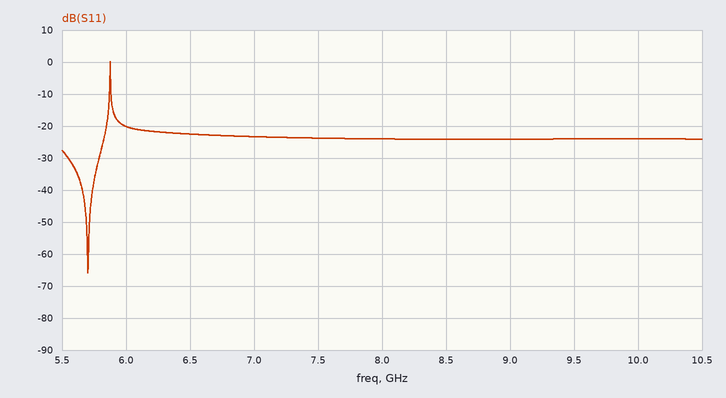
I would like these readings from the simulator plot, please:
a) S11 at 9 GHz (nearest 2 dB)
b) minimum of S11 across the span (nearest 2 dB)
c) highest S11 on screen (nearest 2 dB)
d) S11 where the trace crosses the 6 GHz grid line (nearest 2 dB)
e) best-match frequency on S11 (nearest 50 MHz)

-24 dB
-66 dB
0 dB
-20 dB
5.70 GHz
